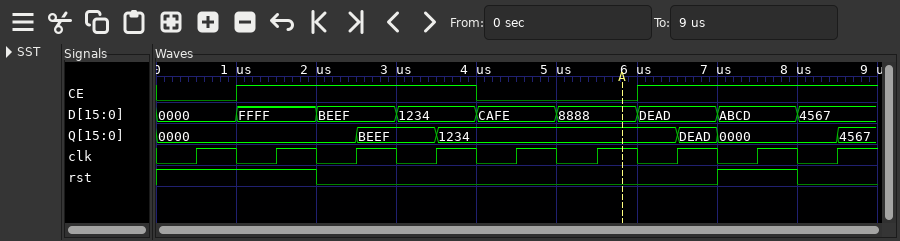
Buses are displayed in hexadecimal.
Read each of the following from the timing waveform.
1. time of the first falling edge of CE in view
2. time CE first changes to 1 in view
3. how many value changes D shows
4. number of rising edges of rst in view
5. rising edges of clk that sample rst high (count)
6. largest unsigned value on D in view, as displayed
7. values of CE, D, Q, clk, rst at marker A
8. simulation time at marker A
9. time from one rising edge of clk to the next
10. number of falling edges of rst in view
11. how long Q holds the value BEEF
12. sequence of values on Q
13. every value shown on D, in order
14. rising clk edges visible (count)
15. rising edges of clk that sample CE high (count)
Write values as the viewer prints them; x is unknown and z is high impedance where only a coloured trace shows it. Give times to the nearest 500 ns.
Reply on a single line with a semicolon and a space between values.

4000 ns; 1000 ns; 8; 1; 3; FFFF; CE=0, D=8888, Q=1234, clk=1, rst=0; 6000 ns; 1000 ns; 2; 1000 ns; 0000, BEEF, 1234, DEAD, 0000, 4567; 0000, FFFF, BEEF, 1234, CAFE, 8888, DEAD, ABCD, 4567; 9; 6
